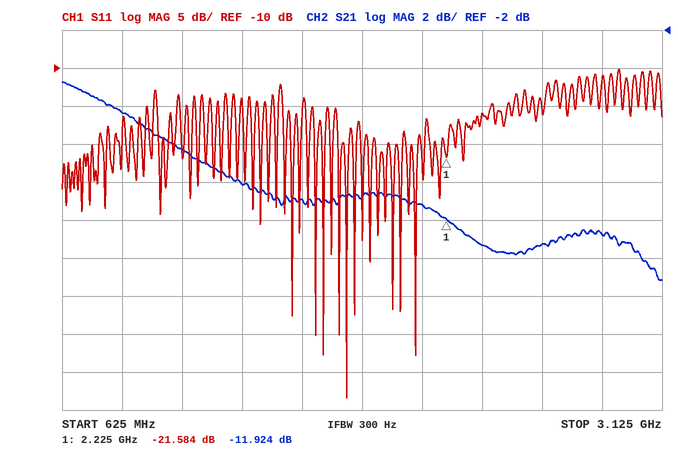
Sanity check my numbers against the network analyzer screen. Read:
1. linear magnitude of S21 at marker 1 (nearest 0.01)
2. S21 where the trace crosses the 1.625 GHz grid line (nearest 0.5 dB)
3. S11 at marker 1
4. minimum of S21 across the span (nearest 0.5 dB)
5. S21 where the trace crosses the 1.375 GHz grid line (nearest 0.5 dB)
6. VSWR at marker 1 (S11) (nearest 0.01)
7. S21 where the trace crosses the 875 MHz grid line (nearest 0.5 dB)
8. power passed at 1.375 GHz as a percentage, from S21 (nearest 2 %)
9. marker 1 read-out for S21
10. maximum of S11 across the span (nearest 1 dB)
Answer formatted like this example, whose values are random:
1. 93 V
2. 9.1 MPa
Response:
1. 0.25
2. -11.0 dB
3. -21.584 dB
4. -15.0 dB
5. -10.0 dB
6. 1.18
7. -6.5 dB
8. 10 %
9. -11.924 dB
10. -10 dB
